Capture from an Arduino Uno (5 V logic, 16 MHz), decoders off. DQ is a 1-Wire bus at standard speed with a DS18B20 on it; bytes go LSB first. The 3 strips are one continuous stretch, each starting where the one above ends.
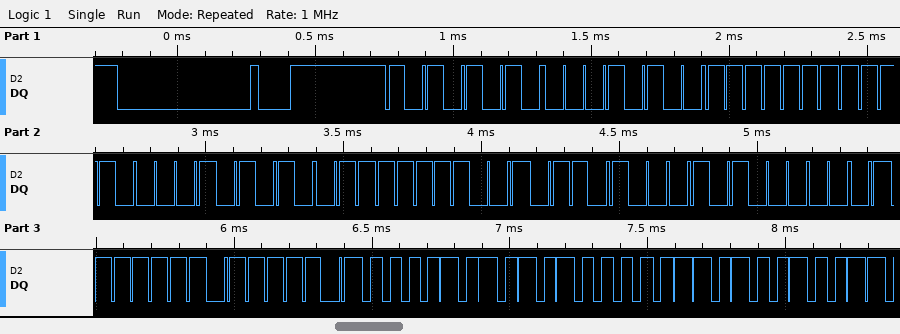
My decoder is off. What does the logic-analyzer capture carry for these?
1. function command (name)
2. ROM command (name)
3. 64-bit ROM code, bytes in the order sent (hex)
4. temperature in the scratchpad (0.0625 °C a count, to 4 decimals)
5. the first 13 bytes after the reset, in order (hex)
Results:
Read Scratchpad
Match ROM
28 FF 87 CA 9F 16 05 FE
85.0000 °C
55 28 FF 87 CA 9F 16 05 FE BE 50 05 4B
